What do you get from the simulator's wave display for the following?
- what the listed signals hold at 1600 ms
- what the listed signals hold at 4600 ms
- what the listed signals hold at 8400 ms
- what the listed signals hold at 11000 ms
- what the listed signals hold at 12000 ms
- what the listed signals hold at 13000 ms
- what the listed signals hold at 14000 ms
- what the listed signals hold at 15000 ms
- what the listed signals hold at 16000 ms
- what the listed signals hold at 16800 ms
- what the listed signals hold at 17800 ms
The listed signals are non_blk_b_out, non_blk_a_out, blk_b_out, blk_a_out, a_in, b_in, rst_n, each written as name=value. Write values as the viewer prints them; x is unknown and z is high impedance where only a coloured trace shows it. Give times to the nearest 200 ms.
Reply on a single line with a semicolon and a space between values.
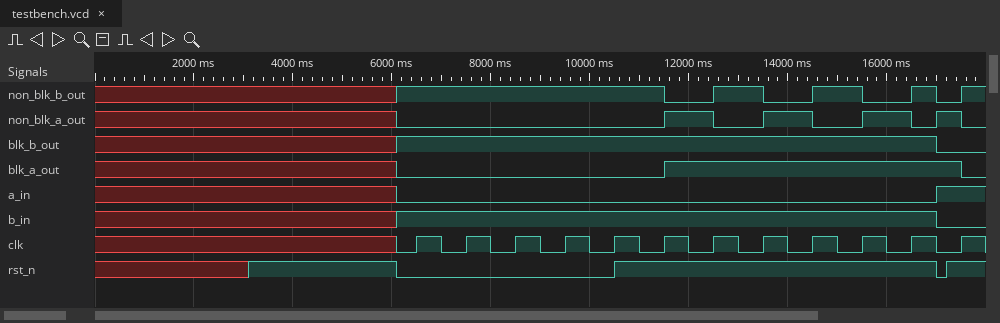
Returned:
non_blk_b_out=x, non_blk_a_out=x, blk_b_out=x, blk_a_out=x, a_in=x, b_in=x, rst_n=x; non_blk_b_out=x, non_blk_a_out=x, blk_b_out=x, blk_a_out=x, a_in=x, b_in=x, rst_n=1; non_blk_b_out=1, non_blk_a_out=0, blk_b_out=1, blk_a_out=0, a_in=0, b_in=1, rst_n=0; non_blk_b_out=1, non_blk_a_out=0, blk_b_out=1, blk_a_out=0, a_in=0, b_in=1, rst_n=1; non_blk_b_out=0, non_blk_a_out=1, blk_b_out=1, blk_a_out=1, a_in=0, b_in=1, rst_n=1; non_blk_b_out=1, non_blk_a_out=0, blk_b_out=1, blk_a_out=1, a_in=0, b_in=1, rst_n=1; non_blk_b_out=0, non_blk_a_out=1, blk_b_out=1, blk_a_out=1, a_in=0, b_in=1, rst_n=1; non_blk_b_out=1, non_blk_a_out=0, blk_b_out=1, blk_a_out=1, a_in=0, b_in=1, rst_n=1; non_blk_b_out=0, non_blk_a_out=1, blk_b_out=1, blk_a_out=1, a_in=0, b_in=1, rst_n=1; non_blk_b_out=1, non_blk_a_out=0, blk_b_out=1, blk_a_out=1, a_in=0, b_in=1, rst_n=1; non_blk_b_out=1, non_blk_a_out=0, blk_b_out=0, blk_a_out=0, a_in=1, b_in=0, rst_n=1
